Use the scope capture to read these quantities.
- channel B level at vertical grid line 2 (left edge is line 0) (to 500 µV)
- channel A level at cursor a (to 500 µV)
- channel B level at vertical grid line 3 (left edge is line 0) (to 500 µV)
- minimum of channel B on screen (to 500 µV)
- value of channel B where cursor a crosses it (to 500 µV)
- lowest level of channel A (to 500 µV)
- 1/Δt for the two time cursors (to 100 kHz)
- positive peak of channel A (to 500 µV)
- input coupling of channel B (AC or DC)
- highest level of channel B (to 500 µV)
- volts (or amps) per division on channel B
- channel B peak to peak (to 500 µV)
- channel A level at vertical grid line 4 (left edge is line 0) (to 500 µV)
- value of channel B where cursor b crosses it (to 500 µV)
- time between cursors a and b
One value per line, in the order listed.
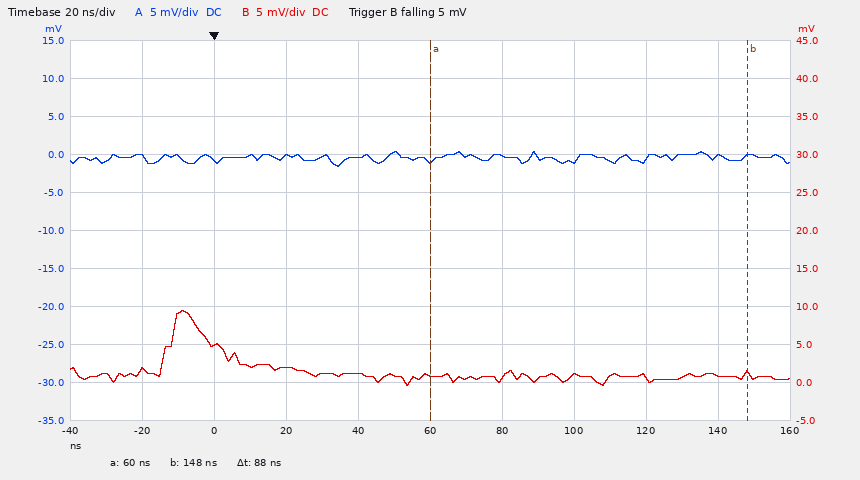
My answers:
5.0 mV
-1.0 mV
2.0 mV
-500 µV
1.0 mV
-1.5 mV
11.4 MHz
500 µV
DC
9.5 mV
5 mV
10.0 mV
-500 µV
1.0 mV
88 ns
